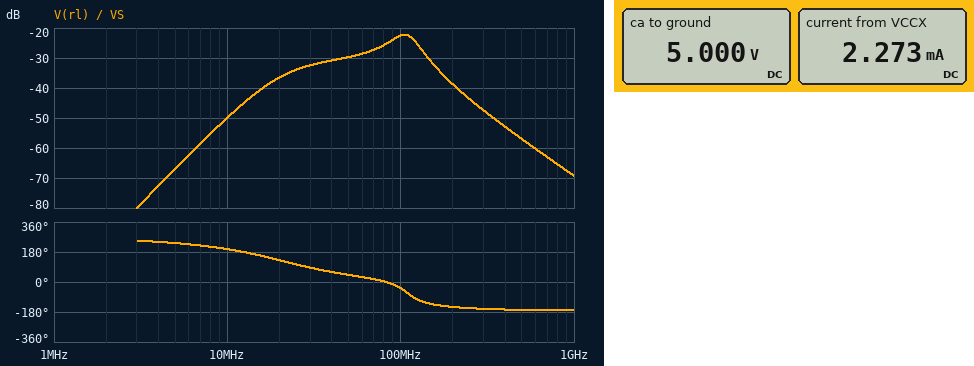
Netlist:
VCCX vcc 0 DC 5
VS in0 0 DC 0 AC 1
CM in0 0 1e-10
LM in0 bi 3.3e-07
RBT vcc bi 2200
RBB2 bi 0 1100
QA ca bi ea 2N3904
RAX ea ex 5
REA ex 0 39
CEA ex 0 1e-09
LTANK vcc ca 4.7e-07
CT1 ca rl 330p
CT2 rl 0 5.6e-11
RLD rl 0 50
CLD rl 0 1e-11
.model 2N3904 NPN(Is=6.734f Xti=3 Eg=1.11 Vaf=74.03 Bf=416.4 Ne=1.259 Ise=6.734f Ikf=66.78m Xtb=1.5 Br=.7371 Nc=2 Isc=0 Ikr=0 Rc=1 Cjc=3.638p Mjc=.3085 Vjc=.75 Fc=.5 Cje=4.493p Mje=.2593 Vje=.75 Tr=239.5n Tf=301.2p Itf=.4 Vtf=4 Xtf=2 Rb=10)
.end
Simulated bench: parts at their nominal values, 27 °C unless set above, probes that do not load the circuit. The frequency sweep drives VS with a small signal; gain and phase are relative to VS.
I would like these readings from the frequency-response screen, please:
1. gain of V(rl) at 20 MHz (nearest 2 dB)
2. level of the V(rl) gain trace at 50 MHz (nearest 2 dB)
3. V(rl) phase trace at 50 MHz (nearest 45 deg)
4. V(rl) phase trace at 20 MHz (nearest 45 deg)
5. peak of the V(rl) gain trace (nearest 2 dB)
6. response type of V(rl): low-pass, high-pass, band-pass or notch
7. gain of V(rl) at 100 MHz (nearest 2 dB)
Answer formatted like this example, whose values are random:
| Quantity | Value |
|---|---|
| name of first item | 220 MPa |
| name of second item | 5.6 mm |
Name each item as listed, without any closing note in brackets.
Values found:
| Quantity | Value |
|---|---|
| gain of V(rl) at 20 MHz | -36 dB |
| level of the V(rl) gain trace at 50 MHz | -30 dB |
| V(rl) phase trace at 50 MHz | 45 deg |
| V(rl) phase trace at 20 MHz | 135 deg |
| peak of the V(rl) gain trace | -22 dB |
| response type of V(rl): low-pass, high-pass, band-pass or notch | band-pass |
| gain of V(rl) at 100 MHz | -22 dB |
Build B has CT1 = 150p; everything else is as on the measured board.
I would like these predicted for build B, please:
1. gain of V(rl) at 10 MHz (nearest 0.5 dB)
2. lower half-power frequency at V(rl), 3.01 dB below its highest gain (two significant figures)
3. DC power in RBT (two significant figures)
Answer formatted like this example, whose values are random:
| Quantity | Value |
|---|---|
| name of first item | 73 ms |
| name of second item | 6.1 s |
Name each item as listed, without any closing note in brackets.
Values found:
| Quantity | Value |
|---|---|
| gain of V(rl) at 10 MHz | -55.0 dB |
| lower half-power frequency at V(rl), 3.01 dB below its highest gain | 82 MHz |
| DC power in RBT | 11 mW |
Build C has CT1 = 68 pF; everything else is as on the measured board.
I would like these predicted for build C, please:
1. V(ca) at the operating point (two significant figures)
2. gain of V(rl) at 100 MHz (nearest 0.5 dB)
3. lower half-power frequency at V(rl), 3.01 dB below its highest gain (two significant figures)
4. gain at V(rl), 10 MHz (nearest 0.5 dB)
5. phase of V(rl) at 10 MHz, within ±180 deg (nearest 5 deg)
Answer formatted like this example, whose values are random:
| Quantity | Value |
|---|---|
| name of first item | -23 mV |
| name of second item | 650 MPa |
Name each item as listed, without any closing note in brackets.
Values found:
| Quantity | Value |
|---|---|
| V(ca) at the operating point | 5.0 V |
| gain of V(rl) at 100 MHz | -22.0 dB |
| lower half-power frequency at V(rl), 3.01 dB below its highest gain | 81 MHz |
| gain at V(rl), 10 MHz | -62.0 dB |
| phase of V(rl) at 10 MHz, within ±180 deg | -115 deg |
